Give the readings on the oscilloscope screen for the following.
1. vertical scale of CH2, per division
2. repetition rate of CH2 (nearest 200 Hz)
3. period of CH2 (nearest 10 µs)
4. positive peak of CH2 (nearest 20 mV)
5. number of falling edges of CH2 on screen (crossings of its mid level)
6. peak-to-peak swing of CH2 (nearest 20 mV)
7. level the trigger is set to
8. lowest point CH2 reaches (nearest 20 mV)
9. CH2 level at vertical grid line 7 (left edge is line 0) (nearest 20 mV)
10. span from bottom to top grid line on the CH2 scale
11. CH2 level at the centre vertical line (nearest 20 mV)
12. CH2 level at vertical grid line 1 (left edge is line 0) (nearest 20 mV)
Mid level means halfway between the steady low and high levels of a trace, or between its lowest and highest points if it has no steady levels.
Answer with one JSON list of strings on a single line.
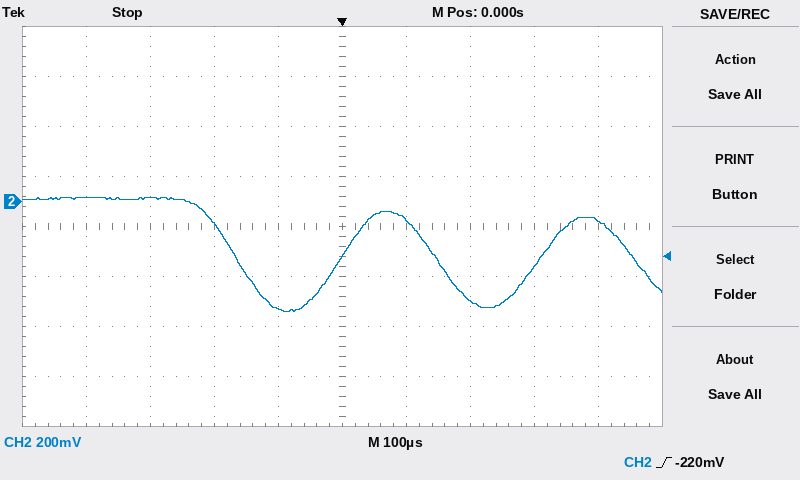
["200 mV", "3.2 kHz", "310 µs", "20 mV", "3", "460 mV", "-220 mV", "-440 mV", "-400 mV", "1.6 V", "-220 mV", "20 mV"]
